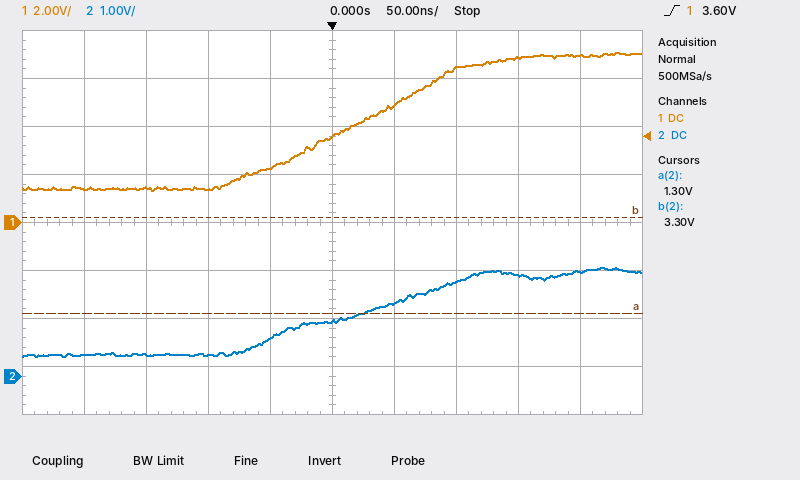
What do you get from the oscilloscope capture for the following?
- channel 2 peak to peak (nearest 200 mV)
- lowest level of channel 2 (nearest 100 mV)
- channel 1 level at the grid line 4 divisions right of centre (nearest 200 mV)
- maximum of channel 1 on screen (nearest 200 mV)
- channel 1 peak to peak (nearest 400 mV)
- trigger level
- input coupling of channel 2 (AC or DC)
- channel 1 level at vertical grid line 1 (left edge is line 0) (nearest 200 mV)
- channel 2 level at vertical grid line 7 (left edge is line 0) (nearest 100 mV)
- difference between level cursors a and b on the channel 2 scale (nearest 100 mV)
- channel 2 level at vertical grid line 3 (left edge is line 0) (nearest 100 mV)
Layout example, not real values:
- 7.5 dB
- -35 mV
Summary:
- 1.8 V
- 400 mV
- 7.0 V
- 7.0 V
- 5.6 V
- 3.60 V
- DC
- 1.4 V
- 2.0 V
- 2.0 V
- 400 mV
